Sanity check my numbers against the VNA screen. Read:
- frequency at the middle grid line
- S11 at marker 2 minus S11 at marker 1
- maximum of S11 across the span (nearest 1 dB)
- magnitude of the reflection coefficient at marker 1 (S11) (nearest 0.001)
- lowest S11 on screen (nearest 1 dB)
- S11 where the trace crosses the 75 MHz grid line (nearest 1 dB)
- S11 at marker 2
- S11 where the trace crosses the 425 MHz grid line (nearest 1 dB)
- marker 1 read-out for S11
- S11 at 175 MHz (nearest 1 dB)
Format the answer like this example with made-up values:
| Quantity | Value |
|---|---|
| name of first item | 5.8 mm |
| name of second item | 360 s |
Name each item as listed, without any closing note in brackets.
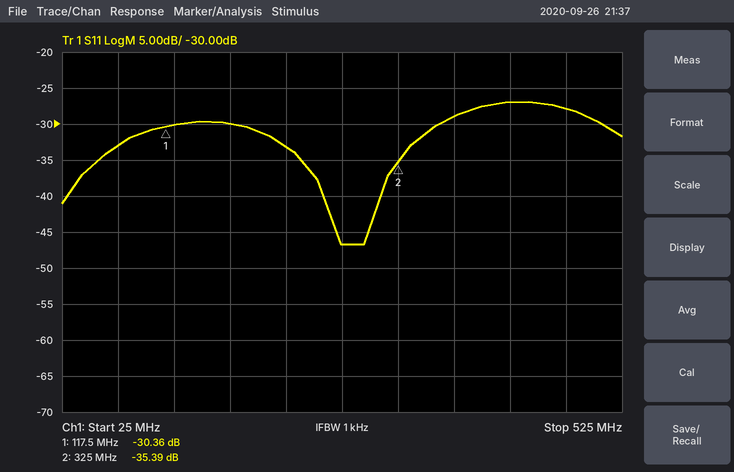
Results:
| Quantity | Value |
|---|---|
| frequency at the middle grid line | 275 MHz |
| S11 at marker 2 minus S11 at marker 1 | -5.03 dB |
| maximum of S11 across the span | -27 dB |
| magnitude of the reflection coefficient at marker 1 (S11) | 0.030 |
| lowest S11 on screen | -47 dB |
| S11 where the trace crosses the 75 MHz grid line | -33 dB |
| S11 at marker 2 | -35.39 dB |
| S11 where the trace crosses the 425 MHz grid line | -27 dB |
| marker 1 read-out for S11 | -30.36 dB |
| S11 at 175 MHz | -30 dB |
